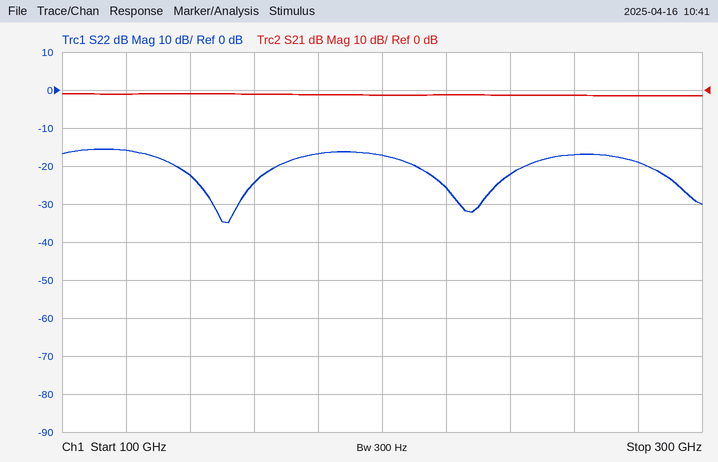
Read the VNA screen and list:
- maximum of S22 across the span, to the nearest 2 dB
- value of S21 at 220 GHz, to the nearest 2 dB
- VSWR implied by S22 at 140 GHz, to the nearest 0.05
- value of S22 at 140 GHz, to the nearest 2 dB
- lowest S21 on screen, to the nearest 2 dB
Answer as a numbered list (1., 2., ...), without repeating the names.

1. -16 dB
2. -2 dB
3. 1.15
4. -22 dB
5. -2 dB
